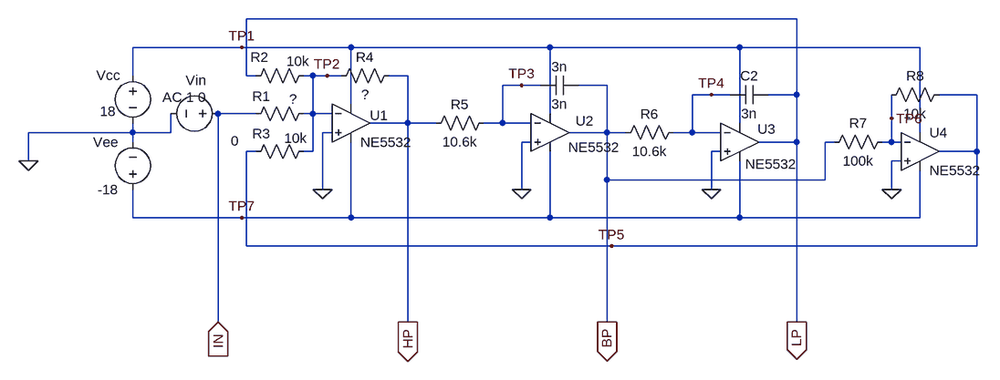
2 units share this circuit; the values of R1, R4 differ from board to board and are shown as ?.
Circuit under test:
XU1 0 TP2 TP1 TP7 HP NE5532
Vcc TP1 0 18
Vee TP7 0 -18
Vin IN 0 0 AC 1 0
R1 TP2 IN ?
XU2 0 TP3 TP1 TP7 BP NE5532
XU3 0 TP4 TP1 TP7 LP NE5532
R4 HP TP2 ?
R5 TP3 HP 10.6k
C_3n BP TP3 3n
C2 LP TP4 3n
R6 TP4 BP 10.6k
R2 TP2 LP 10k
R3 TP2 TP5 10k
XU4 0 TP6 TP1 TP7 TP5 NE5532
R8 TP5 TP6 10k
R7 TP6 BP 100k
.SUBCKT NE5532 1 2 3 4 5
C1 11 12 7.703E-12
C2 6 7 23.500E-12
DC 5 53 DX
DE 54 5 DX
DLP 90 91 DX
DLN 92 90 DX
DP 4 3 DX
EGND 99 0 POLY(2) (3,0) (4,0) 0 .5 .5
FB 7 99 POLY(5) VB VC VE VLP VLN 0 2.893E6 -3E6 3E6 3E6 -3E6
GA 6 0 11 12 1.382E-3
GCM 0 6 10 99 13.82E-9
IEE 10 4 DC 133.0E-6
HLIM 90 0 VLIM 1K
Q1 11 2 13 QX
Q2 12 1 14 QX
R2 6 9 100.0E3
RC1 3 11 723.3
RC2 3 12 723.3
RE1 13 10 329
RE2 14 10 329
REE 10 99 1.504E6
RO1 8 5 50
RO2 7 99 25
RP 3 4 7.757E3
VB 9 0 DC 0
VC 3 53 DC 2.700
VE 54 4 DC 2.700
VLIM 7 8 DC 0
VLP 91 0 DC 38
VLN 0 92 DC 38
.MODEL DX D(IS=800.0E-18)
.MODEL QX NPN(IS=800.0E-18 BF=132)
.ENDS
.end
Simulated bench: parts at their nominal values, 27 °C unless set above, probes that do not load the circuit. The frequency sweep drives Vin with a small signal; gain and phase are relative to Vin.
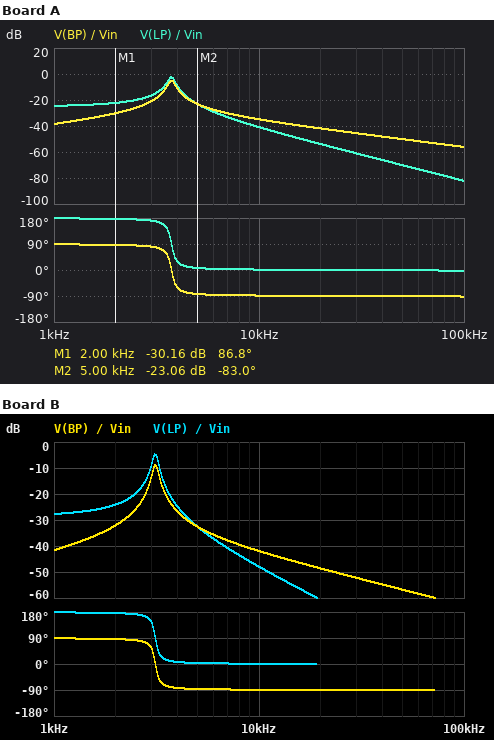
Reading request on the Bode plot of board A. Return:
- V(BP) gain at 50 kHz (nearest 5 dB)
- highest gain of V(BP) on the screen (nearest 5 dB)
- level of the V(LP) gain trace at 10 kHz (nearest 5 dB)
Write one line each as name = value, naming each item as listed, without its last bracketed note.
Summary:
V(BP) gain at 50 kHz = -50 dB
highest gain of V(BP) on the screen = -5 dB
level of the V(LP) gain trace at 10 kHz = -40 dB
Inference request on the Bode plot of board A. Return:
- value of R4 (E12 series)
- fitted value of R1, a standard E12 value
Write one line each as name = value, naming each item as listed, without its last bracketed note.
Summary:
value of R4 = 5.6 kΩ
fitted value of R1, a standard E12 value = 180 kΩ
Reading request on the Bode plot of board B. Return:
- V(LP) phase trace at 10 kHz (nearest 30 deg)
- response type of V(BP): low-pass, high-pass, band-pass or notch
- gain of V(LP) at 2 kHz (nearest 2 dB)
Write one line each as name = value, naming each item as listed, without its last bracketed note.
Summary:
V(LP) phase trace at 10 kHz = 0 deg
response type of V(BP): low-pass, high-pass, band-pass or notch = band-pass
gain of V(LP) at 2 kHz = -24 dB
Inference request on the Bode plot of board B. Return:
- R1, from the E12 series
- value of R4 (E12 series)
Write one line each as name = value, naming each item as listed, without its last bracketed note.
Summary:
R1, from the E12 series = 270 kΩ
value of R4 = 3.9 kΩ
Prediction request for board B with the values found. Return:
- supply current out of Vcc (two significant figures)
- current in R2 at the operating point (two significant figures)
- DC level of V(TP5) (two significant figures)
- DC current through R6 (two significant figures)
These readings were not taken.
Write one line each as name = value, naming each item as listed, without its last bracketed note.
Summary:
supply current out of Vcc = 19 mA
current in R2 at the operating point = 1.3 µA
DC level of V(TP5) = 4.5 mV
DC current through R6 = 500 nA
